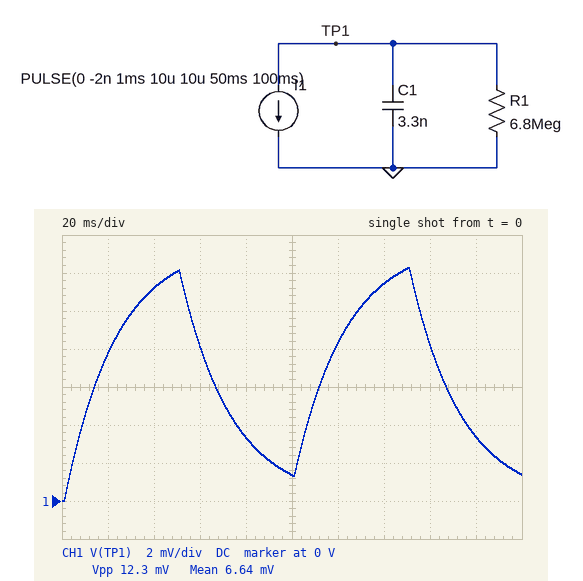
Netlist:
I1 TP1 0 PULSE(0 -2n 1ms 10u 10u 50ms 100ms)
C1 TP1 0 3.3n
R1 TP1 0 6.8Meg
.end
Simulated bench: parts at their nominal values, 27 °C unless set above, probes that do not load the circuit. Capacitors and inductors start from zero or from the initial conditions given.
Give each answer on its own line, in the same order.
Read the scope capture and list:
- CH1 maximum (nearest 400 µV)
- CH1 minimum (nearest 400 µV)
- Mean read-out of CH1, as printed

12.4 mV
0 V
6.64 mV
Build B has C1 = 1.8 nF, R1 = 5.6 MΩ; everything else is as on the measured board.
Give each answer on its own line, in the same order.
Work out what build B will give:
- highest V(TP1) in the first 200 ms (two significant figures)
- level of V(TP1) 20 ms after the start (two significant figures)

11 mV
9.5 mV
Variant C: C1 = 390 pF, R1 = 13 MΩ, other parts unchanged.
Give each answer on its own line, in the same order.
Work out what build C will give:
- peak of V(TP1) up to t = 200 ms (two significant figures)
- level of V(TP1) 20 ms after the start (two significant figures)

26 mV
25 mV
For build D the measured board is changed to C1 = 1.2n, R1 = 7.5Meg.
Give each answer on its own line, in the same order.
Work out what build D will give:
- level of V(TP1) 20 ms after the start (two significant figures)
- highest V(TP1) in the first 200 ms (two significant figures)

13 mV
15 mV
